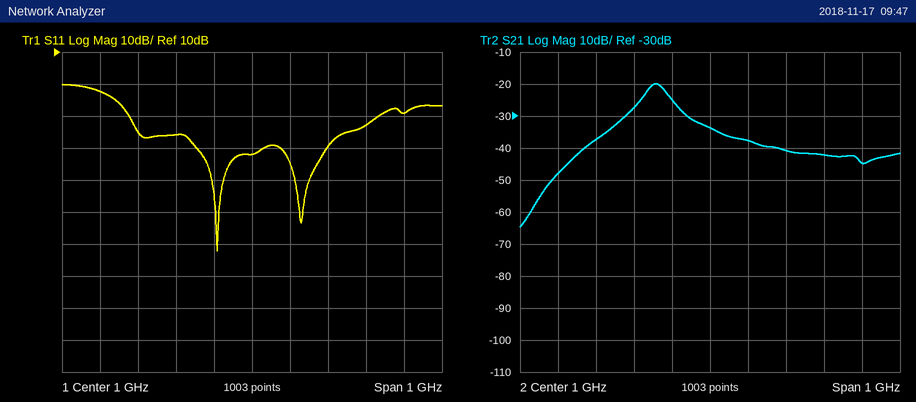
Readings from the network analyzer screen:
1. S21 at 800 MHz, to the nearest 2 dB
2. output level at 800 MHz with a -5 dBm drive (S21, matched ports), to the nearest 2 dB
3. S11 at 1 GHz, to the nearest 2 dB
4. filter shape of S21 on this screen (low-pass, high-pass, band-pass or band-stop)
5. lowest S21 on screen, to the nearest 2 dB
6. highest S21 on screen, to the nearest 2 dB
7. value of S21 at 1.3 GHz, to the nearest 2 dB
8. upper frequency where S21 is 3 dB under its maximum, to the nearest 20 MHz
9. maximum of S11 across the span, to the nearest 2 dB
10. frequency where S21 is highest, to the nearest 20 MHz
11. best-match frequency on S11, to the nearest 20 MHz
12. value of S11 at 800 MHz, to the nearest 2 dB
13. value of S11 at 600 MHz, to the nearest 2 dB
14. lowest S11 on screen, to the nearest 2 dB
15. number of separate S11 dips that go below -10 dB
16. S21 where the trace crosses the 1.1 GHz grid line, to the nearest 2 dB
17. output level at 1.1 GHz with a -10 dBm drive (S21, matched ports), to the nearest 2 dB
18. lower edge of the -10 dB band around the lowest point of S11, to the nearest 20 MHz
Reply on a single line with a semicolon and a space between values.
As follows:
-28 dB; -32 dBm; -22 dB; band-pass; -64 dB; -20 dB; -42 dB; 880 MHz; 0 dB; 860 MHz; 900 MHz; -16 dB; -2 dB; -52 dB; 2; -38 dB; -48 dBm; 680 MHz
